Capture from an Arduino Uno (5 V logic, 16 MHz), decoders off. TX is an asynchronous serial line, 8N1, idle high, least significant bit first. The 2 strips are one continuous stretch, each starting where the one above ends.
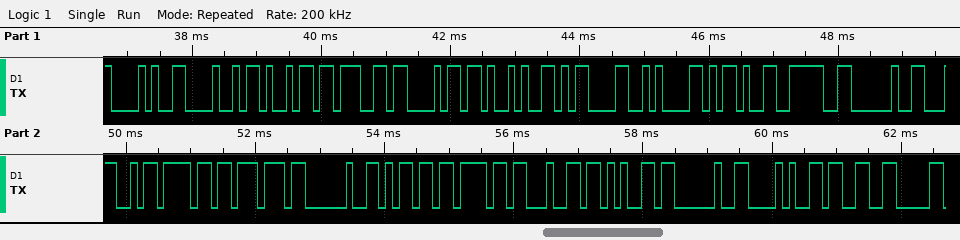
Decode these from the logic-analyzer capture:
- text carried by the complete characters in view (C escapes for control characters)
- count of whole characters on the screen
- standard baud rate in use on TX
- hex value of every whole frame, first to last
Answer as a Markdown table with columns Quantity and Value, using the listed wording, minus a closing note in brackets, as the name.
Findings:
| Quantity | Value |
|---|---|
| text carried by the complete characters in view | "(High)\r\n-> Low mode (3" |
| count of whole characters on the screen | 22 |
| standard baud rate in use on TX | 9600 baud |
| hex value of every whole frame, first to last | 28 48 69 67 68 29 0D 0A 2D 3E 20 4C 6F 77 20 6D 6F 64 65 20 28 33 |
